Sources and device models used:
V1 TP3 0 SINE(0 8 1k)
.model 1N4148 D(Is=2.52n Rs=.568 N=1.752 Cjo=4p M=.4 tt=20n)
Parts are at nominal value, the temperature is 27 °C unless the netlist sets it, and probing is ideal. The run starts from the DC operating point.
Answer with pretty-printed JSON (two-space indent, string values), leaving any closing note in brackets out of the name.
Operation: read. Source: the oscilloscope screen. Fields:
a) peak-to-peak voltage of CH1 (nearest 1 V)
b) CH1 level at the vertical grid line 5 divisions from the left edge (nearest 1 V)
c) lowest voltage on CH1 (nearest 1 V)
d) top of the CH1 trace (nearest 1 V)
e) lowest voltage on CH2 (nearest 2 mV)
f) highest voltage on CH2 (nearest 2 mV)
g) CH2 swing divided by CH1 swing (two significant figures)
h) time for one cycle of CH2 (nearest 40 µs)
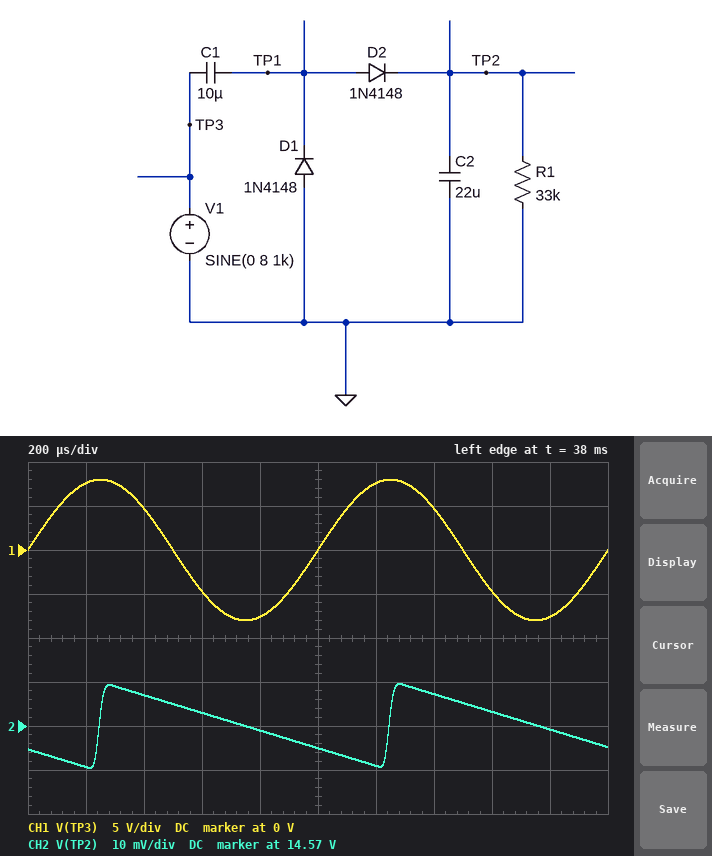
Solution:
{
  "peak-to-peak voltage of CH1": "16 V",
  "CH1 level at the vertical grid line 5 divisions from the left edge": "0 V",
  "lowest voltage on CH1": "-8 V",
  "top of the CH1 trace": "8 V",
  "lowest voltage on CH2": "14.560 V",
  "highest voltage on CH2": "14.580 V",
  "CH2 swing divided by CH1 swing": "0.0012",
  "time for one cycle of CH2": "1.00 ms"
}
